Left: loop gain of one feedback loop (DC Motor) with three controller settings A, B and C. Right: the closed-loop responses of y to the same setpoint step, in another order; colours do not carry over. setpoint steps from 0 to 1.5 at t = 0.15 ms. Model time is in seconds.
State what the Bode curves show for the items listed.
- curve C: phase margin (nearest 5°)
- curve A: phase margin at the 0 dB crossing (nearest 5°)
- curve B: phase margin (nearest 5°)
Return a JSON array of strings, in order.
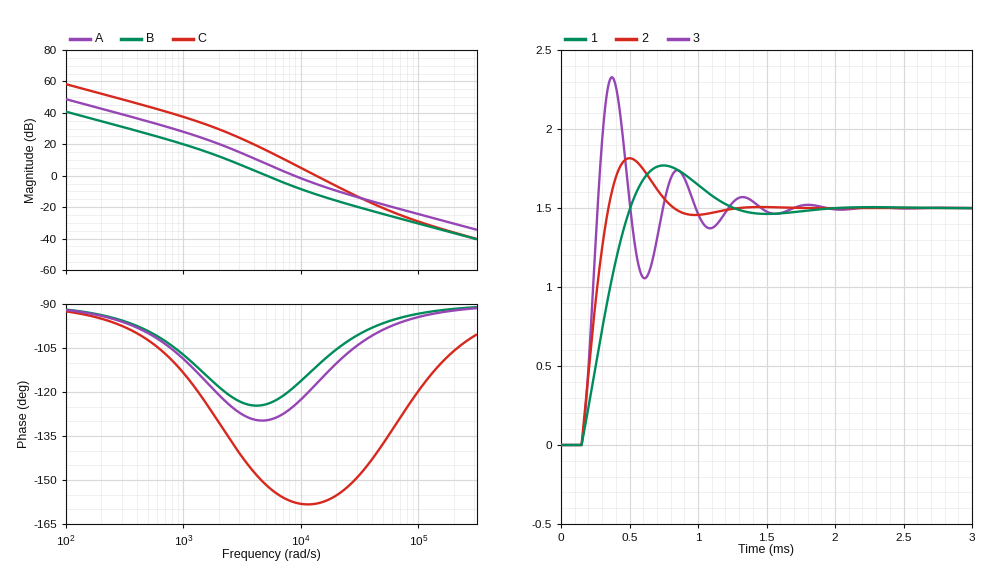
["20°", "55°", "55°"]
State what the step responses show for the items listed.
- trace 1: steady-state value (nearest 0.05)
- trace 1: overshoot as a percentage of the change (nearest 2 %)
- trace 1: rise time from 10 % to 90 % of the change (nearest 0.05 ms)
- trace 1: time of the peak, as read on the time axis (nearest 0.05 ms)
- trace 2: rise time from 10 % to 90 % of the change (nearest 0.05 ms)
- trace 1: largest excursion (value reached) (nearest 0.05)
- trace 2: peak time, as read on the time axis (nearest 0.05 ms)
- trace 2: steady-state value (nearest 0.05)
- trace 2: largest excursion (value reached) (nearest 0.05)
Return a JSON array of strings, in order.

["1.50", "18 %", "0.25 ms", "0.75 ms", "0.15 ms", "1.75", "0.50 ms", "1.50", "1.80"]
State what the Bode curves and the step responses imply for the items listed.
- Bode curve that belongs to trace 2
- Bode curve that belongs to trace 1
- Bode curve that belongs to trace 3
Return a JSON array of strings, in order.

["A", "B", "C"]
